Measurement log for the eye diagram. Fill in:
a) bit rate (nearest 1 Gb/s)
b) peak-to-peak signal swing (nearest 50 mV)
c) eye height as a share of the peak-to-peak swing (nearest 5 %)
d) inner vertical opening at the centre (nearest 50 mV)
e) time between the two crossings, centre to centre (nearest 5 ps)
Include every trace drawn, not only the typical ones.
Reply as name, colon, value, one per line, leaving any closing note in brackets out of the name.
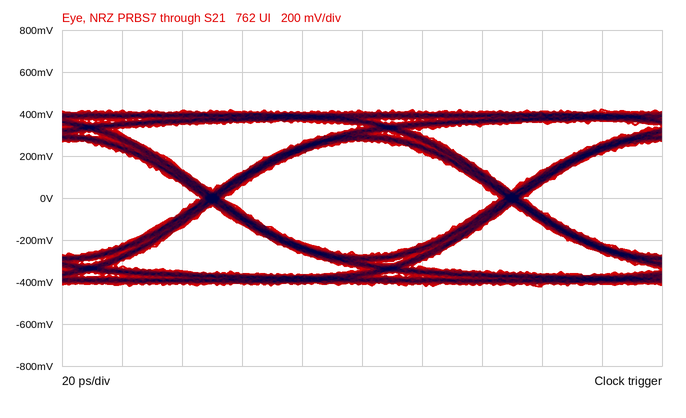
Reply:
bit rate: 10 Gb/s
peak-to-peak signal swing: 850 mV
eye height as a share of the peak-to-peak swing: 65 %
inner vertical opening at the centre: 550 mV
time between the two crossings, centre to centre: 100 ps
